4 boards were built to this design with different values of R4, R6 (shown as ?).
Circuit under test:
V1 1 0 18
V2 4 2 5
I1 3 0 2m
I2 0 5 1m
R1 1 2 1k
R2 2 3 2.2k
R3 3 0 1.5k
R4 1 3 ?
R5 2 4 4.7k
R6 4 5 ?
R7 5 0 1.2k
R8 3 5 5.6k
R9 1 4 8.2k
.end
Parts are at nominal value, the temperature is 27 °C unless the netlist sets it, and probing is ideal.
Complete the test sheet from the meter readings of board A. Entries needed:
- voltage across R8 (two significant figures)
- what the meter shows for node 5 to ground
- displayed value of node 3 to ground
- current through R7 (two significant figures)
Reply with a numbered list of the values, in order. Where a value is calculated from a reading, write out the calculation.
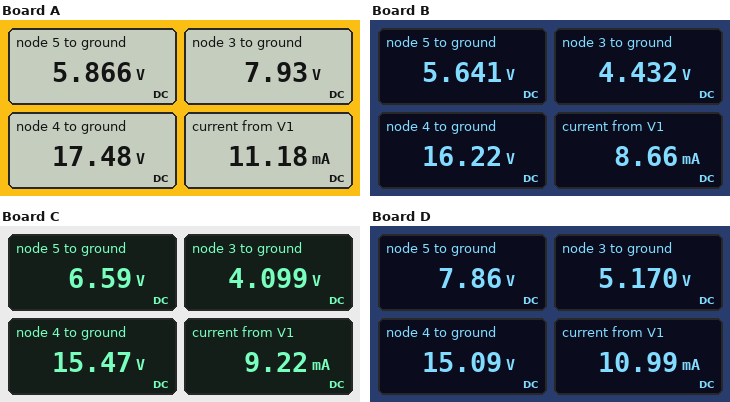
1. 7.93 V - 5.866 V = 2.1 V
2. 5.866 V
3. 7.93 V
4. (5.866 V) / 1.2 kΩ = 4.9 mA
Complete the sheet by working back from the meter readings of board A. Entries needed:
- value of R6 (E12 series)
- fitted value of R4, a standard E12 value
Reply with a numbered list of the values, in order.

1. 3.3 kΩ
2. 1.8 kΩ
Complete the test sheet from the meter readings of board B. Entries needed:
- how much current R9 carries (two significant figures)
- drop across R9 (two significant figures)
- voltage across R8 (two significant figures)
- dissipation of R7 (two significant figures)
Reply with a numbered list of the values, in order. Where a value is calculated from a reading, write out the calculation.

1. (18 V - 16.22 V) / 8.2 kΩ = 220 µA
2. 18 V - 16.22 V = 1.8 V
3. 5.641 V - 4.432 V = 1.2 V
4. (5.641 V)^2 / 1.2 kΩ = 27 mW
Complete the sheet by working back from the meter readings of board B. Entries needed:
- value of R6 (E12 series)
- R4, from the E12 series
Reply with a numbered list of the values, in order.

1. 2.7 kΩ
2. 8.2 kΩ
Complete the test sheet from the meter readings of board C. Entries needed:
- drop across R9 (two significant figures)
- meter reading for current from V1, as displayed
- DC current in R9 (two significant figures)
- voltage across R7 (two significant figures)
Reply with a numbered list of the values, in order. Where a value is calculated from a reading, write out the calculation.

1. 18 V - 15.47 V = 2.5 V
2. 9.22 mA
3. (18 V - 15.47 V) / 8.2 kΩ = 310 µA
4. 6.59 V = 6.6 V
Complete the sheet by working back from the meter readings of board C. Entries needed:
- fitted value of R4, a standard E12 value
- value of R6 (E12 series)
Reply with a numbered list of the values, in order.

1. 10 kΩ
2. 1.8 kΩ
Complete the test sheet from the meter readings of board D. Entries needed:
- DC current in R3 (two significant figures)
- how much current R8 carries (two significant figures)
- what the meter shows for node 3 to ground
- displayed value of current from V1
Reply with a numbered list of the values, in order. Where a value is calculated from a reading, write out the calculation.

1. (5.17 V) / 1.5 kΩ = 3.4 mA
2. (7.86 V - 5.17 V) / 5.6 kΩ = 480 µA
3. 5.170 V
4. 10.99 mA
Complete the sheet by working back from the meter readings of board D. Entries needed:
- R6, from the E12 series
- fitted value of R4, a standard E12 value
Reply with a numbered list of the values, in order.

1. 1.2 kΩ
2. 4.7 kΩ
